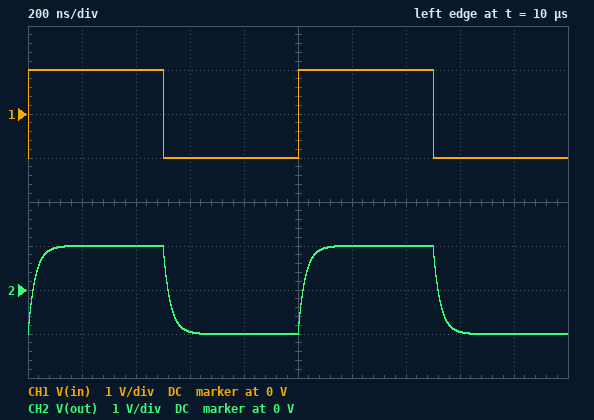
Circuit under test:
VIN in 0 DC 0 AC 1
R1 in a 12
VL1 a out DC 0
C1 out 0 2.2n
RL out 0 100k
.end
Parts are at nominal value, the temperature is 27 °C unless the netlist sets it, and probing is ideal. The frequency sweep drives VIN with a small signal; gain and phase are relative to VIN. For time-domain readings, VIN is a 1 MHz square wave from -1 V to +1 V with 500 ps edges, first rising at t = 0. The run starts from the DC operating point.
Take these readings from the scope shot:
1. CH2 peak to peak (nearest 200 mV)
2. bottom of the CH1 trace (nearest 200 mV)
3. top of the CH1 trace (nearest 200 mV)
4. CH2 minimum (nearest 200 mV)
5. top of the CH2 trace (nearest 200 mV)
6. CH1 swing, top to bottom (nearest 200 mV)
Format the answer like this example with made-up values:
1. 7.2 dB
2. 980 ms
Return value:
1. 2.0 V
2. -1.0 V
3. 1.0 V
4. -1.0 V
5. 1.0 V
6. 2.0 V
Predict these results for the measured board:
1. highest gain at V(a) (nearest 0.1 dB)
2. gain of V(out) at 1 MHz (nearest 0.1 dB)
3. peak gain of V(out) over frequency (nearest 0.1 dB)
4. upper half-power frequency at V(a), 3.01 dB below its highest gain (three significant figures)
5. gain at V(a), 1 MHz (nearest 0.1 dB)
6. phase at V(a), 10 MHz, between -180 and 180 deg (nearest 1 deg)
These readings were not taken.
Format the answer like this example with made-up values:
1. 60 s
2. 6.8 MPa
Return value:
1. 0 dB
2. -0.1 dB
3. 0 dB
4. 6.03 MHz
5. -0.1 dB
6. -59 deg
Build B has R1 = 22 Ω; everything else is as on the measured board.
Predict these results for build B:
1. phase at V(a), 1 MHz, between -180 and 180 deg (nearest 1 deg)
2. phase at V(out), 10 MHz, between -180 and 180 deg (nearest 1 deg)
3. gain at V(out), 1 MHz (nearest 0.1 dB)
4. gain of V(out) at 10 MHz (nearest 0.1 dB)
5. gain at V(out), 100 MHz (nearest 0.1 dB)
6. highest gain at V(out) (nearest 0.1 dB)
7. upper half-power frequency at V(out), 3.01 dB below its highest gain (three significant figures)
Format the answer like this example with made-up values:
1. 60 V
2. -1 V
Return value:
1. -17 deg
2. -72 deg
3. -0.4 dB
4. -10.1 dB
5. -29.7 dB
6. 0 dB
7. 3.29 MHz
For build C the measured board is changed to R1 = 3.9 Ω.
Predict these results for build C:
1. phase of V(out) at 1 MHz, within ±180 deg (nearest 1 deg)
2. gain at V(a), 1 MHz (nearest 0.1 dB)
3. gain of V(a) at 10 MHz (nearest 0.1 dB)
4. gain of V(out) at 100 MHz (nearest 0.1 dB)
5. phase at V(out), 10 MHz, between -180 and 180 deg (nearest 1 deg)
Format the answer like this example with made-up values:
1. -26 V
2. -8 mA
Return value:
1. -3 deg
2. 0 dB
3. -1.1 dB
4. -14.8 dB
5. -28 deg
